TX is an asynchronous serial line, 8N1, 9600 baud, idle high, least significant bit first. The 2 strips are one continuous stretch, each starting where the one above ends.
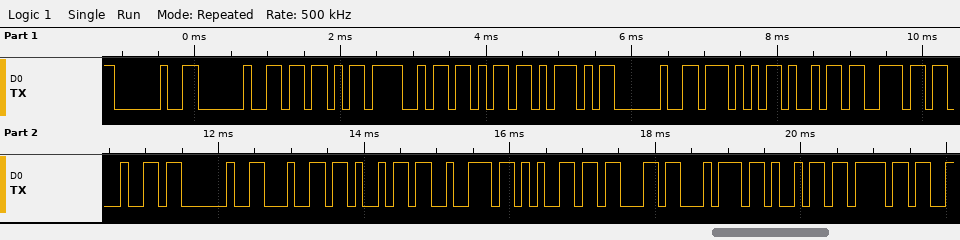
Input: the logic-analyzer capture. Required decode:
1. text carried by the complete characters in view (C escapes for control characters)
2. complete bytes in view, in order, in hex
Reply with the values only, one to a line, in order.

"  [Ok] Wind directio"
20 20 5B 4F 6B 5D 20 57 69 6E 64 20 64 69 72 65 63 74 69 6F
